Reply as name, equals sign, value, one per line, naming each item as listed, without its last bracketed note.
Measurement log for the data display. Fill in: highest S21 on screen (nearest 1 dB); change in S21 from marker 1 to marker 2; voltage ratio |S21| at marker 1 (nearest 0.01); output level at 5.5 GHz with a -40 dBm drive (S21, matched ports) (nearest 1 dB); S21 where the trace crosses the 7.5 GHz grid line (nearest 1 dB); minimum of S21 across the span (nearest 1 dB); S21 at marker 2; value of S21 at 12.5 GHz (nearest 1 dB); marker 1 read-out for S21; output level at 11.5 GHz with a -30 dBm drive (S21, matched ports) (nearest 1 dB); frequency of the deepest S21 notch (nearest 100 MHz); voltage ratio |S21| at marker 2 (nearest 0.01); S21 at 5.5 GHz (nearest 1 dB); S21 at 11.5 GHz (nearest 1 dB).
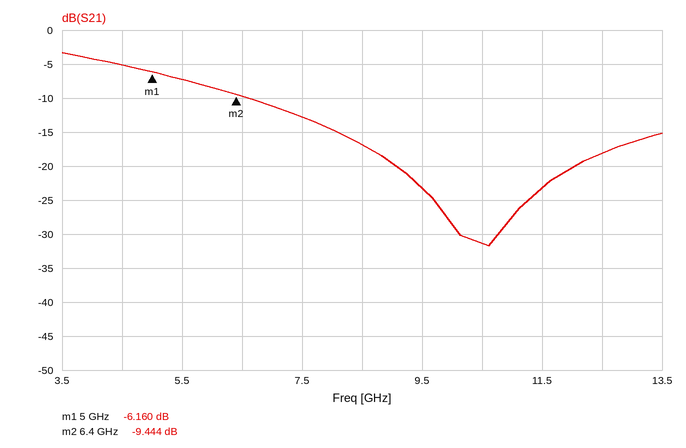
highest S21 on screen = -3 dB
change in S21 from marker 1 to marker 2 = -3.284 dB
voltage ratio |S21| at marker 1 = 0.49
output level at 5.5 GHz with a -40 dBm drive (S21, matched ports) = -47 dBm
S21 where the trace crosses the 7.5 GHz grid line = -13 dB
minimum of S21 across the span = -32 dB
S21 at marker 2 = -9.444 dB
value of S21 at 12.5 GHz = -18 dB
marker 1 read-out for S21 = -6.160 dB
output level at 11.5 GHz with a -30 dBm drive (S21, matched ports) = -53 dBm
frequency of the deepest S21 notch = 10.6 GHz
voltage ratio |S21| at marker 2 = 0.34
S21 at 5.5 GHz = -7 dB
S21 at 11.5 GHz = -23 dB
